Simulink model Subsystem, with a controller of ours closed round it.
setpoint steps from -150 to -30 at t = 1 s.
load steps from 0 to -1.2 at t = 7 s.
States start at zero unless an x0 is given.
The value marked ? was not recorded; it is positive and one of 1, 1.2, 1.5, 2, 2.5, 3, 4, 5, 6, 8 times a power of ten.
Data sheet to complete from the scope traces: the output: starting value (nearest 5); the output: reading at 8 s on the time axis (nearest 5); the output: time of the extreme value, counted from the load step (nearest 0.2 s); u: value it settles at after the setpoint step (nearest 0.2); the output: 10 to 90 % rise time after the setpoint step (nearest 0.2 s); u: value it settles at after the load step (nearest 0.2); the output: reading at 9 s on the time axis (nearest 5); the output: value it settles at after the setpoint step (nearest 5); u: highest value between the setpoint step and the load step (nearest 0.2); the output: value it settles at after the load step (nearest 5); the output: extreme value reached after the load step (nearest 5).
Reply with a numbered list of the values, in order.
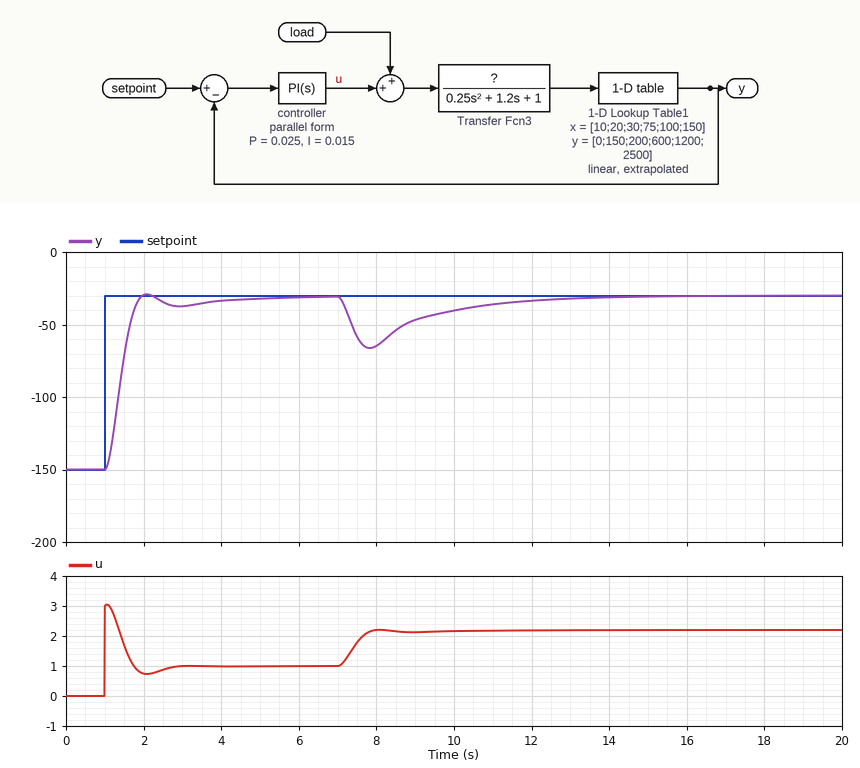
1. -150
2. -65
3. 0.8 s
4. 1.0
5. 0.6 s
6. 2.2
7. -45
8. -30
9. 3.0
10. -30
11. -65
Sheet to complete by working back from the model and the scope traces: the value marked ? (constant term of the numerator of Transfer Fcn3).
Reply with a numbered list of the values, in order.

1. 8
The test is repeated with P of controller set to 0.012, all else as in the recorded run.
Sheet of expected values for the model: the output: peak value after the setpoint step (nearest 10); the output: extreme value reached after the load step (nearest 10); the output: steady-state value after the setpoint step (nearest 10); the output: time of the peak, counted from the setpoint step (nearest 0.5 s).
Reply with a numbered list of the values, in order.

1. -20
2. -80
3. -30
4. 2.0 s
